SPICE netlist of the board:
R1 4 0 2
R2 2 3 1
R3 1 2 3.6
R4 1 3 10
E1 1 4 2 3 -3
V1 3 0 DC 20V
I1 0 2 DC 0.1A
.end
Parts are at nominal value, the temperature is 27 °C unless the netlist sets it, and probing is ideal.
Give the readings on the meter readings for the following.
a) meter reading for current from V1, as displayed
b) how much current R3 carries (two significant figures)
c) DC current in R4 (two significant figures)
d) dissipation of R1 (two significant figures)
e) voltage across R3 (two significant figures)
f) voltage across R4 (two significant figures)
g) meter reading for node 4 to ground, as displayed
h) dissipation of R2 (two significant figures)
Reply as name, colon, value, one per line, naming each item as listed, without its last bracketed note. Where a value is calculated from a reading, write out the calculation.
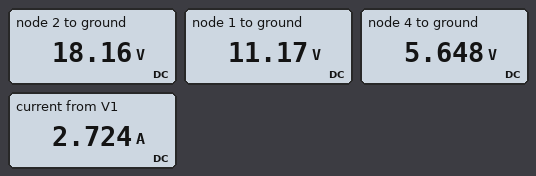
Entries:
meter reading for current from V1, as displayed: 2.724 A
how much current R3 carries: (18.16 V - 11.17 V) / 3.6 Ω = 1.9 A
DC current in R4: (20 V - 11.17 V) / 10 Ω = 880 mA
dissipation of R1: (5.648 V)^2 / 2 Ω = 16 W
voltage across R3: 18.16 V - 11.17 V = 7.0 V
voltage across R4: 20 V - 11.17 V = 8.8 V
meter reading for node 4 to ground, as displayed: 5.648 V
dissipation of R2: (20 V - 18.16 V)^2 / 1 Ω = 3.4 W
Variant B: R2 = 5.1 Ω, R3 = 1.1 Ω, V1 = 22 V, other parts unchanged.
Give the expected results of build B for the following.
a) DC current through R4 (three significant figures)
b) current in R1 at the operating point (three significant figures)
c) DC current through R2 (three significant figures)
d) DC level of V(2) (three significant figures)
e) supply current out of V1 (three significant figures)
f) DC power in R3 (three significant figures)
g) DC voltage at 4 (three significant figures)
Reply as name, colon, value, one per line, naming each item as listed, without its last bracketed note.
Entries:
DC current through R4: 554 mA
current in R1 at the operating point: 1.53 A
DC current through R2: 876 mA
DC level of V(2): 17.5 V
supply current out of V1: 1.43 A
DC power in R3: 1.05 W
DC voltage at 4: 3.06 V
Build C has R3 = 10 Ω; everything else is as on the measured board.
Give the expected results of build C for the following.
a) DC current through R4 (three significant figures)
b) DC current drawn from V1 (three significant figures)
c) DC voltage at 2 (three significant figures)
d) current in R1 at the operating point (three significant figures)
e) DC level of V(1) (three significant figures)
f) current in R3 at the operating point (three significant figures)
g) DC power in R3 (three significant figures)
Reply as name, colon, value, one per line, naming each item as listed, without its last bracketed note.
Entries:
DC current through R4: 1.22 A
DC current drawn from V1: 2.25 A
DC voltage at 2: 19.0 V
current in R1 at the operating point: 2.35 A
DC level of V(1): 7.76 V
current in R3 at the operating point: 1.12 A
DC power in R3: 12.6 W
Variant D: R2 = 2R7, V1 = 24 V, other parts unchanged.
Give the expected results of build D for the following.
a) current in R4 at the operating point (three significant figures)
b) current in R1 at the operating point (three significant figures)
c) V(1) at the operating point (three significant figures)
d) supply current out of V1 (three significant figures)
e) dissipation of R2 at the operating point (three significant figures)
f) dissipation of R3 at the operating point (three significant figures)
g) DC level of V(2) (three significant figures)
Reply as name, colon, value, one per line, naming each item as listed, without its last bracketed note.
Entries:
current in R4 at the operating point: 870 mA
current in R1 at the operating point: 2.29 A
V(1) at the operating point: 15.3 V
supply current out of V1: 2.19 A
dissipation of R2 at the operating point: 4.73 W
dissipation of R3 at the operating point: 7.29 W
DC level of V(2): 20.4 V
